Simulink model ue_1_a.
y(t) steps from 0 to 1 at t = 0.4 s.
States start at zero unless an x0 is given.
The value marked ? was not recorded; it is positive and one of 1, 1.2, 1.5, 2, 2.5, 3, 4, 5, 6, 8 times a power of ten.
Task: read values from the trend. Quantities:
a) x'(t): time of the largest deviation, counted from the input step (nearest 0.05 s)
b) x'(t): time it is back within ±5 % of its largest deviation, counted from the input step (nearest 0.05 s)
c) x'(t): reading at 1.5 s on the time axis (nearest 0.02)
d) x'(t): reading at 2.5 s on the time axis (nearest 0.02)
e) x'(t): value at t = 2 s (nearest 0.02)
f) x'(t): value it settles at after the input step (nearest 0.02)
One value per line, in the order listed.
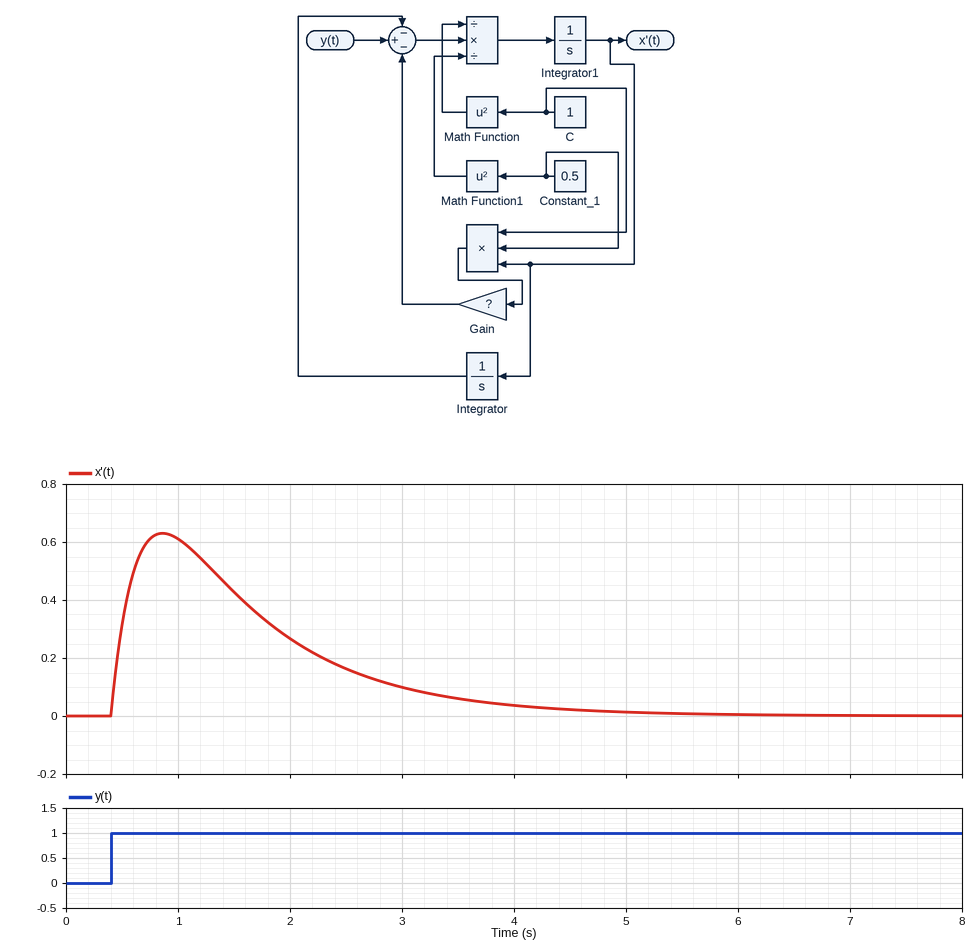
0.45 s
3.75 s
0.42
0.16
0.26
0.00
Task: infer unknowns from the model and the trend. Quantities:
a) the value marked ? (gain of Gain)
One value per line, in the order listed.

2.5
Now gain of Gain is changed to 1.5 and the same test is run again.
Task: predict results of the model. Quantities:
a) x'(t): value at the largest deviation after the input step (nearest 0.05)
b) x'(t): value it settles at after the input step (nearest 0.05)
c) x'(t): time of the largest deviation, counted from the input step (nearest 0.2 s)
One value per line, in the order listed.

0.90
0.00
0.6 s
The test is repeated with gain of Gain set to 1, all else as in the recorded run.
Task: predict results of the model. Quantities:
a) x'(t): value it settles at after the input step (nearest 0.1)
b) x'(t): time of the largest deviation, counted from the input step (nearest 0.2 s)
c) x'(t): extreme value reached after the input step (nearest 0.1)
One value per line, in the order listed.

0.0
0.6 s
1.1
